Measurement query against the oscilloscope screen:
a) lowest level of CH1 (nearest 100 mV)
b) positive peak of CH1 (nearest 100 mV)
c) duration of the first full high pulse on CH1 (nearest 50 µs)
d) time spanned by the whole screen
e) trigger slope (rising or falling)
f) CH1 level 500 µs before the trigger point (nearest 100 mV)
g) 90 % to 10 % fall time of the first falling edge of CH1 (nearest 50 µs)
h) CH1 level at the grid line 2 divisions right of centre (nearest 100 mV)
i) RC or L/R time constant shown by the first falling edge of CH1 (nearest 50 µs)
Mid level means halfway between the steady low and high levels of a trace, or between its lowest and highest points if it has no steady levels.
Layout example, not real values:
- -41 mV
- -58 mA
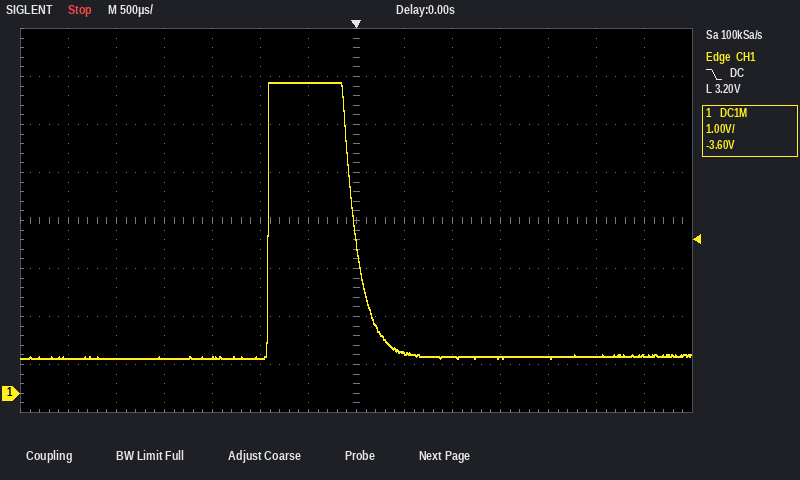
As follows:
- 700 mV
- 6.5 V
- 900 µs
- 7 ms
- falling
- 6.5 V
- 350 µs
- 800 mV
- 150 µs
